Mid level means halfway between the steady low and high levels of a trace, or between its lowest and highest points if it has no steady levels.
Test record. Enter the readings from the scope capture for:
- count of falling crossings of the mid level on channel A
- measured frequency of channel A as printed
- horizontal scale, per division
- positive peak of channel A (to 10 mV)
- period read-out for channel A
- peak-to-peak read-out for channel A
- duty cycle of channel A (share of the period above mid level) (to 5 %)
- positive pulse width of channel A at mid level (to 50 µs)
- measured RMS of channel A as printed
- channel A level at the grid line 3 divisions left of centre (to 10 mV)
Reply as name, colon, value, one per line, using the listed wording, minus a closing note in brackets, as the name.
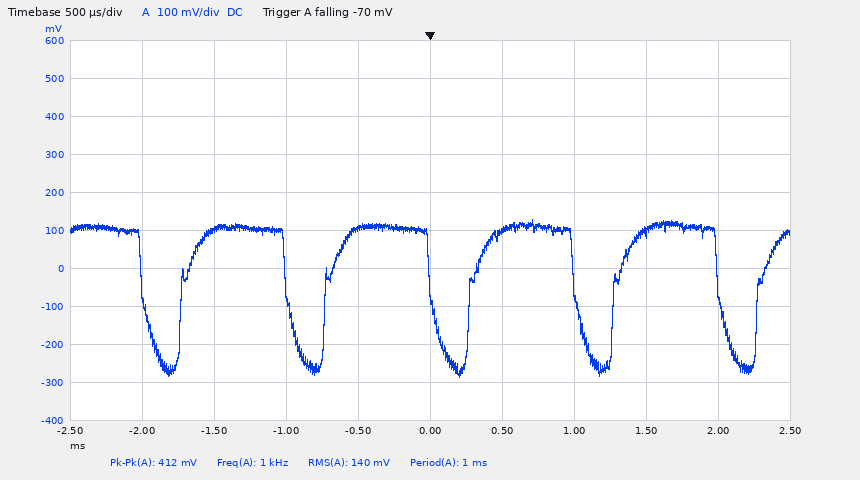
count of falling crossings of the mid level on channel A: 5
measured frequency of channel A as printed: 1 kHz
horizontal scale, per division: 500 µs
positive peak of channel A: 130 mV
period read-out for channel A: 1 ms
peak-to-peak read-out for channel A: 412 mV
duty cycle of channel A (share of the period above mid level): 75 %
positive pulse width of channel A at mid level: 750 µs
measured RMS of channel A as printed: 140 mV
channel A level at the grid line 3 divisions left of centre: 100 mV
